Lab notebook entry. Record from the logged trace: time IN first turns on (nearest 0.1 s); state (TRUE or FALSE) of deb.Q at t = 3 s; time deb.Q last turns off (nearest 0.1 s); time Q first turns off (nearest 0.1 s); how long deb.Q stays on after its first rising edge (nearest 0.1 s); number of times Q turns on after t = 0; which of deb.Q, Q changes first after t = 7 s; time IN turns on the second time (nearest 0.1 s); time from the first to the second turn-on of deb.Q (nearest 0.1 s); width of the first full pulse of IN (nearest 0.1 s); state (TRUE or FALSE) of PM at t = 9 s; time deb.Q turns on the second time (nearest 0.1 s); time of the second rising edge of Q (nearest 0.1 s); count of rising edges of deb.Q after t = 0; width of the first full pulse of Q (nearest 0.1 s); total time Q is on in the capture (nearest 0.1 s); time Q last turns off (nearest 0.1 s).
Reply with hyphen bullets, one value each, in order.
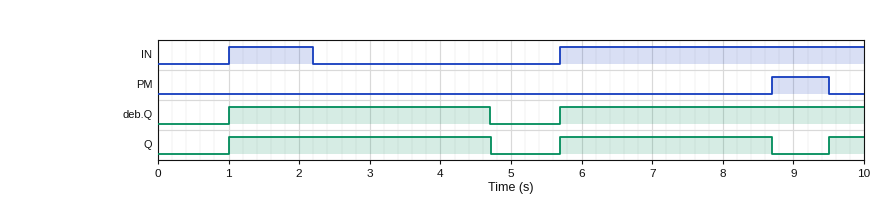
- 1.0 s
- TRUE
- 4.7 s
- 4.7 s
- 3.7 s
- 3
- Q
- 5.7 s
- 4.7 s
- 1.2 s
- TRUE
- 5.7 s
- 5.7 s
- 2
- 3.7 s
- 7.2 s
- 8.7 s
